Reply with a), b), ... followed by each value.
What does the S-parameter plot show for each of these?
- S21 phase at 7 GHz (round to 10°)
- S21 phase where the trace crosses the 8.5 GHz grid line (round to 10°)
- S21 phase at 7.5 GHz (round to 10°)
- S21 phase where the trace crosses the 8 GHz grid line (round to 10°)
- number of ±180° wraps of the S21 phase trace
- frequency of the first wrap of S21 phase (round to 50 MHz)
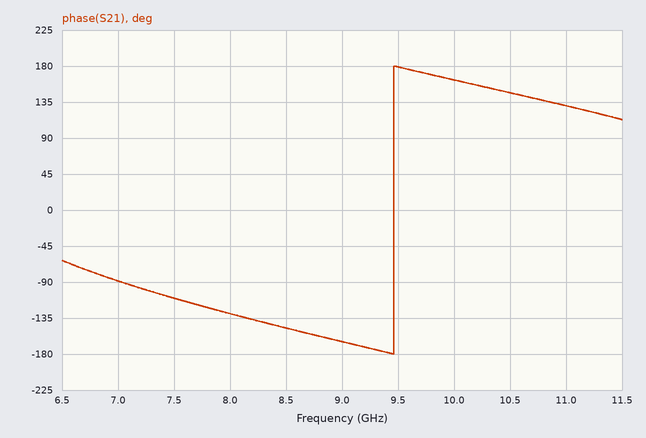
a) -90°
b) -150°
c) -110°
d) -130°
e) 1
f) 9.45 GHz
